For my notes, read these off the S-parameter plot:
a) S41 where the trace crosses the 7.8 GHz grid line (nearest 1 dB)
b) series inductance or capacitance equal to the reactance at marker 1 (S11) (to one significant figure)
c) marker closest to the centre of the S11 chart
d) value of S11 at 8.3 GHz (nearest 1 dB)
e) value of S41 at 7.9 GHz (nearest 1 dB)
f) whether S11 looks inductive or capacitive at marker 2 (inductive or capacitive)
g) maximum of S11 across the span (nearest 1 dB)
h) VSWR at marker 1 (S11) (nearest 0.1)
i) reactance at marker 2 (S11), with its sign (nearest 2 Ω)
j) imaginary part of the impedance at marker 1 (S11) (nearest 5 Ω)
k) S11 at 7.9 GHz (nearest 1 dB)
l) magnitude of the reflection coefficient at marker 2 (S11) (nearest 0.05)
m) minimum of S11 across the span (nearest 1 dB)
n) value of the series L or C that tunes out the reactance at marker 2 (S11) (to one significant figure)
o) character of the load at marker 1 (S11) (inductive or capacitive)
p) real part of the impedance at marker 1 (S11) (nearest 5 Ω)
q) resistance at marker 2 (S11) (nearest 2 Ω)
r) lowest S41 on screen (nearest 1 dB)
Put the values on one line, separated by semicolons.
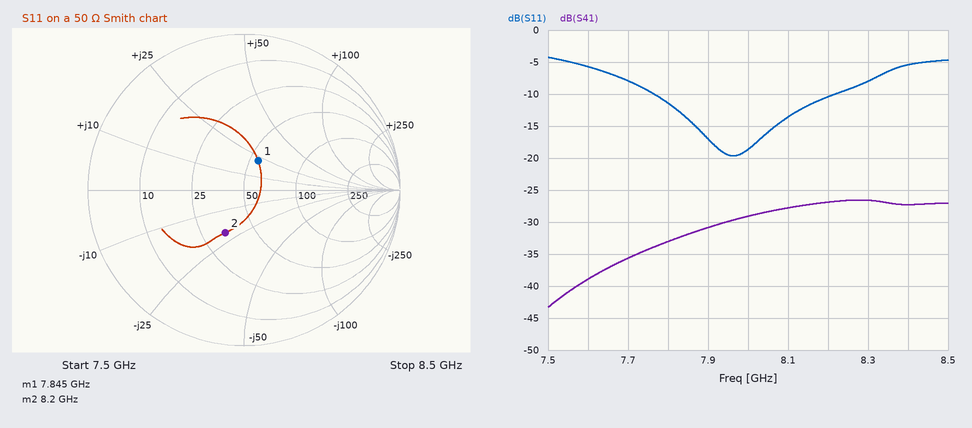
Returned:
-33 dB; 400 pH; marker 1; -8 dB; -31 dB; capacitive; -4 dB; 1.5; -20 Ω; +20 Ω; -17 dB; 0.30; -20 dB; 400 pH; inductive; 55 Ω; 34 Ω; -43 dB
